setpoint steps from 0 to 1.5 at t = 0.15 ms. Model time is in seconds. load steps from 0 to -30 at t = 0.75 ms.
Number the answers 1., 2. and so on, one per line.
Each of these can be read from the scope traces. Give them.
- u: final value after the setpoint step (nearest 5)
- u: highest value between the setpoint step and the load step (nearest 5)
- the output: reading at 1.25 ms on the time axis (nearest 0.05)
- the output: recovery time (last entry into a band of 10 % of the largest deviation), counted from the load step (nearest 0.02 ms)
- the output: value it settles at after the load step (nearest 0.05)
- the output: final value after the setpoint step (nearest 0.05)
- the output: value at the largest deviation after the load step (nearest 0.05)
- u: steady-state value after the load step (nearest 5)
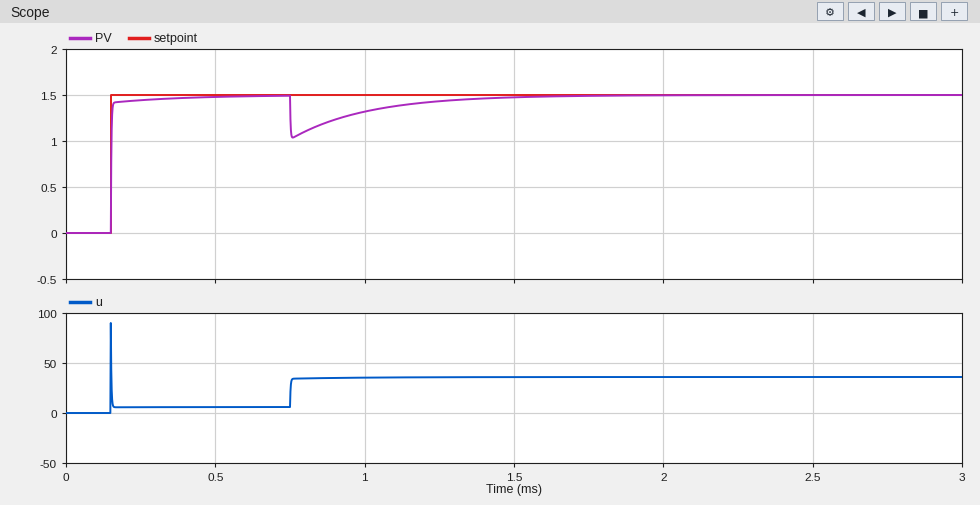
1. 5
2. 90
3. 1.45
4. 0.60 ms
5. 1.50
6. 1.50
7. 1.05
8. 35
